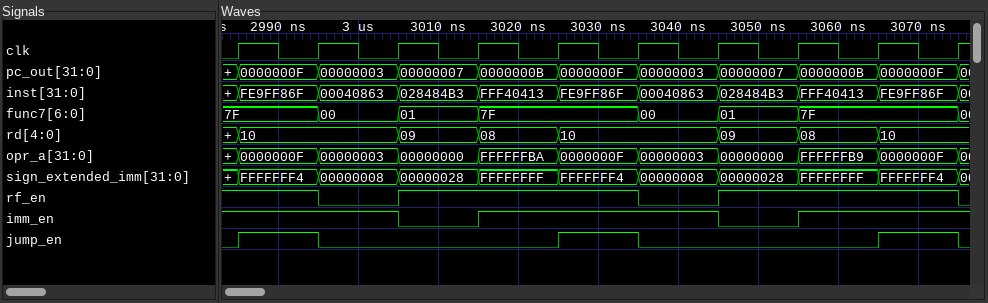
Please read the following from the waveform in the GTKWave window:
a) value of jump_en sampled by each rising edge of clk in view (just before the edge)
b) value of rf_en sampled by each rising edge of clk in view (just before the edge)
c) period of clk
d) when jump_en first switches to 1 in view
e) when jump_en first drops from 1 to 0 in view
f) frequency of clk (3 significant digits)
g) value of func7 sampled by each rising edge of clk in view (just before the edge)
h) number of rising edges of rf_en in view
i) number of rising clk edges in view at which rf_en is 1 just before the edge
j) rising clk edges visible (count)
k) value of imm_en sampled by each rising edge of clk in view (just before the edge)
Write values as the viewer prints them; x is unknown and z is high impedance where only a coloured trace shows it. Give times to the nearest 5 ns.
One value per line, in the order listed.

0 1 0 0 0 1 0 0 0 1
1 1 0 1 1 1 0 1 1 1
10 ns
2985 ns
2995 ns
100 MHz
7F, 7F, 00, 01, 7F, 7F, 00, 01, 7F, 7F
2
8
10
1 1 1 0 1 1 1 0 1 1
